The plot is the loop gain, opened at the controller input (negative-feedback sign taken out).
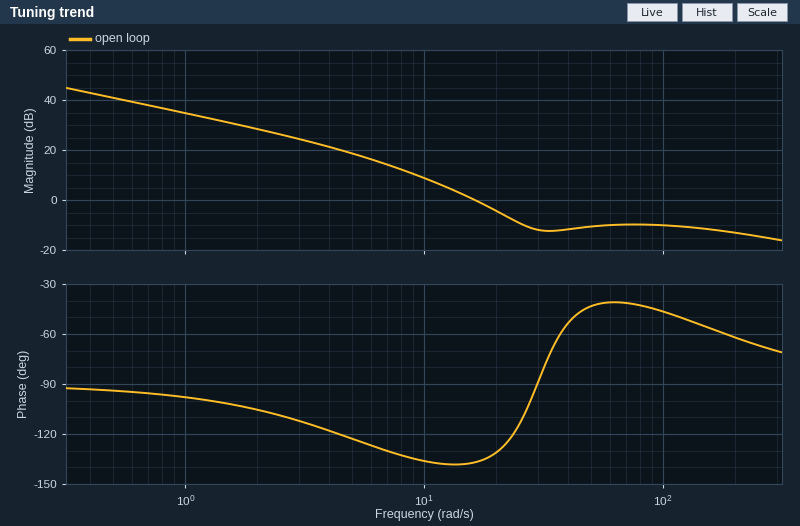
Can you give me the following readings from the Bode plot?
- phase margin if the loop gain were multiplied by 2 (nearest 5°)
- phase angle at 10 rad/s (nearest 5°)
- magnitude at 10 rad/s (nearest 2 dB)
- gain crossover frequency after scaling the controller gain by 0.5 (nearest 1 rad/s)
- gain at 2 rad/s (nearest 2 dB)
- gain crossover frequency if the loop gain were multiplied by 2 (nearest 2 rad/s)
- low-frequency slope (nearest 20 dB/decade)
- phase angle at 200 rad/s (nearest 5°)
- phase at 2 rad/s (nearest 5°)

55°
-135°
8 dB
12 rad/s
28 dB
22 rad/s
-20 dB/decade
-60°
-105°
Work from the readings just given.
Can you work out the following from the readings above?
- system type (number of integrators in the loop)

1
